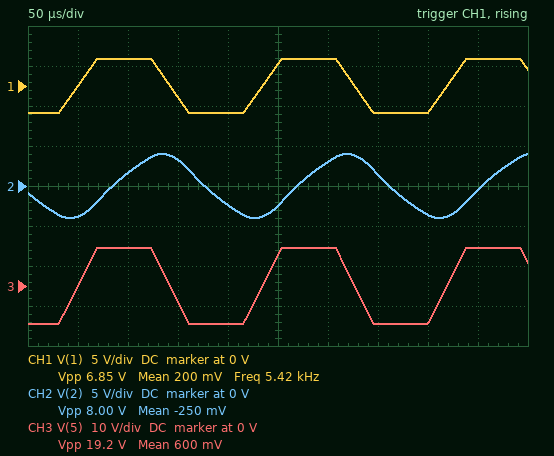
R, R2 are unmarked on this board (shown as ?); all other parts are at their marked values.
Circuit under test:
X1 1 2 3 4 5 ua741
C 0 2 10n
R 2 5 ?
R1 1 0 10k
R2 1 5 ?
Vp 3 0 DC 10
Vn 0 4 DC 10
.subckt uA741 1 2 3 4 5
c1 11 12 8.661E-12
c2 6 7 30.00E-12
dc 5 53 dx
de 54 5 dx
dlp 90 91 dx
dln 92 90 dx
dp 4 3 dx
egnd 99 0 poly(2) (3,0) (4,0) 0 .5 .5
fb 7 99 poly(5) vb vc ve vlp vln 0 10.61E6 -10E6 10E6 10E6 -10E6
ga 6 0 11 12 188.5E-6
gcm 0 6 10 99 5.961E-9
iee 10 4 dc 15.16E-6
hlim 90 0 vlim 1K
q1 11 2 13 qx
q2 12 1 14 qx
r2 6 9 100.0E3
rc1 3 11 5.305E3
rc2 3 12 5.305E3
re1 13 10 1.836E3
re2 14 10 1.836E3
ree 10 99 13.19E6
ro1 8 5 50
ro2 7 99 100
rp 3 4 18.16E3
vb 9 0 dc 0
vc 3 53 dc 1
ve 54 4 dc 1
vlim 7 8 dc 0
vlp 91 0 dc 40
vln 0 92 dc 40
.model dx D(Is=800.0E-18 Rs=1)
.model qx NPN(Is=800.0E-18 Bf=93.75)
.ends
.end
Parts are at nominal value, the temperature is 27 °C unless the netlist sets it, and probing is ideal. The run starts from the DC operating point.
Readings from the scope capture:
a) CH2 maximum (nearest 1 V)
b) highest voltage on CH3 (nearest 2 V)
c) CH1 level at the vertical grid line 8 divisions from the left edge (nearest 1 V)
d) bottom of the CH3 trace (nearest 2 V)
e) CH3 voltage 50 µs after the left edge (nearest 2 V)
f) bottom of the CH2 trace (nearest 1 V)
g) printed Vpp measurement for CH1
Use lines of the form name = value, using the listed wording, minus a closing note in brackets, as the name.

CH2 maximum = 4 V
highest voltage on CH3 = 10 V
CH1 level at the vertical grid line 8 divisions from the left edge = -3 V
bottom of the CH3 trace = -10 V
CH3 voltage 50 µs after the left edge = 0 V
bottom of the CH2 trace = -4 V
printed Vpp measurement for CH1 = 6.85 V
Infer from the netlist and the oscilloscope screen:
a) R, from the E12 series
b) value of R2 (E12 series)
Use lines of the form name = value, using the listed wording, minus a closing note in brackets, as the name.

R, from the E12 series = 8.2 kΩ
value of R2 = 18 kΩ
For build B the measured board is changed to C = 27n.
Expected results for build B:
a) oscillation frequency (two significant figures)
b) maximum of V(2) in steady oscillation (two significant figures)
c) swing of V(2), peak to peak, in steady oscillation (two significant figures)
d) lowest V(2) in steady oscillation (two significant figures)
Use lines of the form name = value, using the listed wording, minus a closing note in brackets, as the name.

oscillation frequency = 2.5 kHz
maximum of V(2) in steady oscillation = 3.7 V
swing of V(2), peak to peak, in steady oscillation = 7.3 V
lowest V(2) in steady oscillation = -3.7 V
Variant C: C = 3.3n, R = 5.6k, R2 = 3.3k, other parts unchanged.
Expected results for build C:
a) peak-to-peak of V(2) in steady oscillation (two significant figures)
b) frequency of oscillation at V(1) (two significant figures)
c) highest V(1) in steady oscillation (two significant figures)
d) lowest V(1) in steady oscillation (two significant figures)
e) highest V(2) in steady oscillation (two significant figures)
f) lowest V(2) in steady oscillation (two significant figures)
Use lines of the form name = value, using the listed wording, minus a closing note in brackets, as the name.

peak-to-peak of V(2) in steady oscillation = 15 V
frequency of oscillation at V(1) = 8.0 kHz
highest V(1) in steady oscillation = 7.2 V
lowest V(1) in steady oscillation = -7.2 V
highest V(2) in steady oscillation = 7.7 V
lowest V(2) in steady oscillation = -7.7 V
